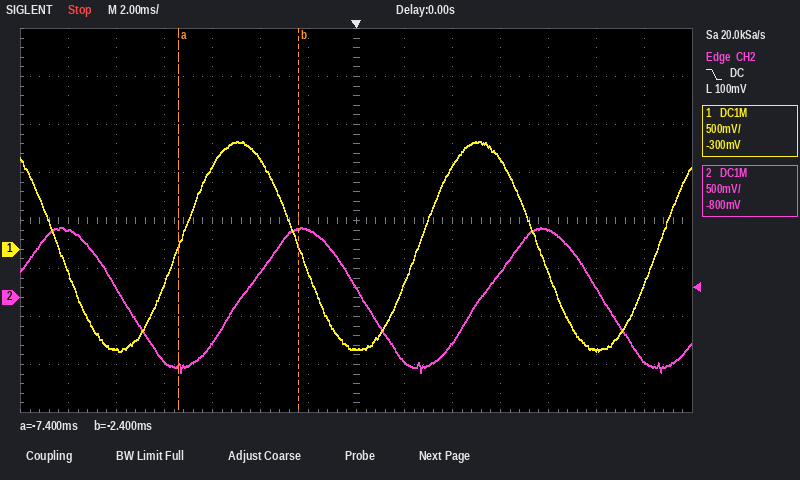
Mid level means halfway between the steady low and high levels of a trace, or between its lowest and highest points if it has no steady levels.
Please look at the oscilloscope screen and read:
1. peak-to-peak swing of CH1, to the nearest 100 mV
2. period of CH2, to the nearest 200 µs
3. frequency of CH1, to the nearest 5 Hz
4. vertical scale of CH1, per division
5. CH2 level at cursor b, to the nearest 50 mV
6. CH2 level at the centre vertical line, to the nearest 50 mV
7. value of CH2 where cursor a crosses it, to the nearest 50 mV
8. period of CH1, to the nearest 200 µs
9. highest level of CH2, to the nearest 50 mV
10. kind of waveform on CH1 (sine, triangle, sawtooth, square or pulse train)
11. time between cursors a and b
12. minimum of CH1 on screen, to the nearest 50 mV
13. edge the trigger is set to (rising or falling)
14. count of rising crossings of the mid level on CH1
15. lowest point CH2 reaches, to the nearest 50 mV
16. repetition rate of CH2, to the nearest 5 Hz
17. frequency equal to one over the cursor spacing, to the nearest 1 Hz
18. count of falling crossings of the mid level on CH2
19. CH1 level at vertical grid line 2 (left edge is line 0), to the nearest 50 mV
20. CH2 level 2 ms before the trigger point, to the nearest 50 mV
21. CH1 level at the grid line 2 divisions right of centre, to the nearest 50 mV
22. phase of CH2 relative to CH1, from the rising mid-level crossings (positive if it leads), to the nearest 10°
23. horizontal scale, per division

2.20 V
10.0 ms
100 Hz
500 mV
700 mV
100 mV
-750 mV
10.0 ms
750 mV
sine
5.0 ms
-1.05 V
falling
3
-800 mV
100 Hz
200 Hz
3
-1.05 V
700 mV
850 mV
-90°
2 ms
